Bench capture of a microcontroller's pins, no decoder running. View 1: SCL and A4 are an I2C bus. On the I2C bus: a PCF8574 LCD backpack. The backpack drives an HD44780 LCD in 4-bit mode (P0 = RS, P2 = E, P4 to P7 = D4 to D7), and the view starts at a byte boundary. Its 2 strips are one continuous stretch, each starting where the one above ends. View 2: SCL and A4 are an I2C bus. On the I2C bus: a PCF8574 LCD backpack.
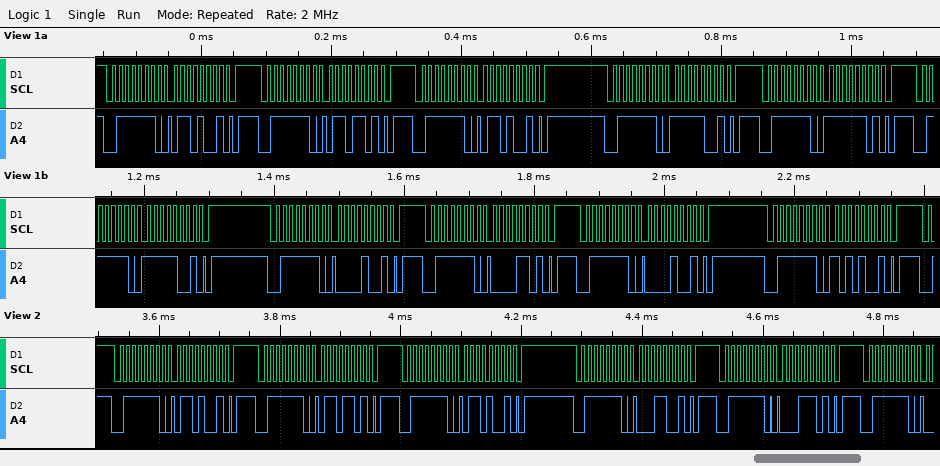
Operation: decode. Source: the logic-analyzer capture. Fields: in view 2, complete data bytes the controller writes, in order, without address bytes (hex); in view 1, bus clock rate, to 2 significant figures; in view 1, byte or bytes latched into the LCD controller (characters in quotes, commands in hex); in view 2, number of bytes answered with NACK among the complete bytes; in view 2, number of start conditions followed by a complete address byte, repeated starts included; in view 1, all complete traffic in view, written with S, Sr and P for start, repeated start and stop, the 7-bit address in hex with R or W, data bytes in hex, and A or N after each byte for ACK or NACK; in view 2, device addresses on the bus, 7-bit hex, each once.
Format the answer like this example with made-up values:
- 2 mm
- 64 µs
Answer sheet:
- 69 6D 69 19 1D
- 100 kHz
- 'o'
- 0
- 6
- S 3FW A 69 A P S 3FW A 6D A P S 3FW A 69 A P S 3FW A F9 A P S 3FW A FD A P S 3FW A F9 A P S 3FW A 09 A P S 3FW A 0D A P S 3FW A 09 A P S 3FW A A9 A P
- 0x3F
